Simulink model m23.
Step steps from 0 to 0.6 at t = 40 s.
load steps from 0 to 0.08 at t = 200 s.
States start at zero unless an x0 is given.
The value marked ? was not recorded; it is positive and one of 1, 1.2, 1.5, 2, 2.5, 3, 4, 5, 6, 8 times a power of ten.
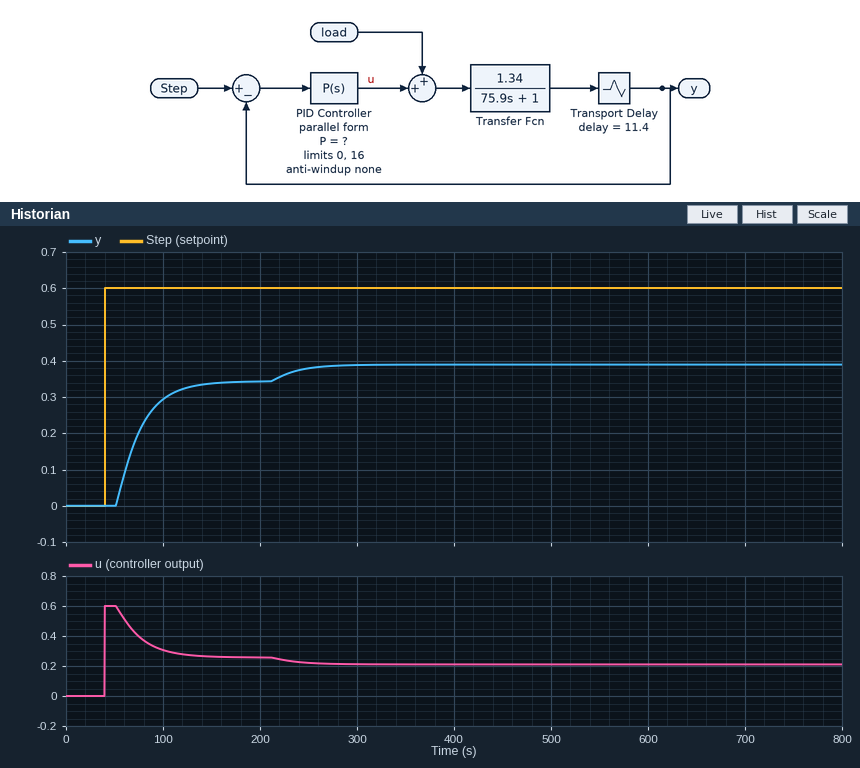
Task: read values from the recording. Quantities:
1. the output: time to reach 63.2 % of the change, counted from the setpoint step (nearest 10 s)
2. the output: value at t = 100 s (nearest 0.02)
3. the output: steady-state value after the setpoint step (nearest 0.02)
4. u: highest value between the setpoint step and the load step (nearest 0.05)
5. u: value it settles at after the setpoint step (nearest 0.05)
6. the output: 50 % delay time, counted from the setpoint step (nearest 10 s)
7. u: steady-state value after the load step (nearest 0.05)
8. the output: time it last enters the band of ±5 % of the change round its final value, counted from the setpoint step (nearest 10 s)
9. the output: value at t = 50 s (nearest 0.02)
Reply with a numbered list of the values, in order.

1. 40 s
2. 0.30
3. 0.34
4. 0.60
5. 0.25
6. 30 s
7. 0.20
8. 90 s
9. 0.00
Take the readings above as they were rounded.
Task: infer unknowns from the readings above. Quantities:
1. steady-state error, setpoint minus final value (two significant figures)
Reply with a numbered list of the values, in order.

1. 0.26
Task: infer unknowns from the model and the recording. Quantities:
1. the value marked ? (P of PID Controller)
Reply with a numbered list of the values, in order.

1. 1
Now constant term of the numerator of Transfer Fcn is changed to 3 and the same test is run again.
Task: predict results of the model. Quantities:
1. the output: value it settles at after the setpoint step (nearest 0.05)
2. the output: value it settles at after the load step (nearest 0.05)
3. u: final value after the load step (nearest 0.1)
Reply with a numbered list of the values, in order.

1. 0.45
2. 0.50
3. 0.1
